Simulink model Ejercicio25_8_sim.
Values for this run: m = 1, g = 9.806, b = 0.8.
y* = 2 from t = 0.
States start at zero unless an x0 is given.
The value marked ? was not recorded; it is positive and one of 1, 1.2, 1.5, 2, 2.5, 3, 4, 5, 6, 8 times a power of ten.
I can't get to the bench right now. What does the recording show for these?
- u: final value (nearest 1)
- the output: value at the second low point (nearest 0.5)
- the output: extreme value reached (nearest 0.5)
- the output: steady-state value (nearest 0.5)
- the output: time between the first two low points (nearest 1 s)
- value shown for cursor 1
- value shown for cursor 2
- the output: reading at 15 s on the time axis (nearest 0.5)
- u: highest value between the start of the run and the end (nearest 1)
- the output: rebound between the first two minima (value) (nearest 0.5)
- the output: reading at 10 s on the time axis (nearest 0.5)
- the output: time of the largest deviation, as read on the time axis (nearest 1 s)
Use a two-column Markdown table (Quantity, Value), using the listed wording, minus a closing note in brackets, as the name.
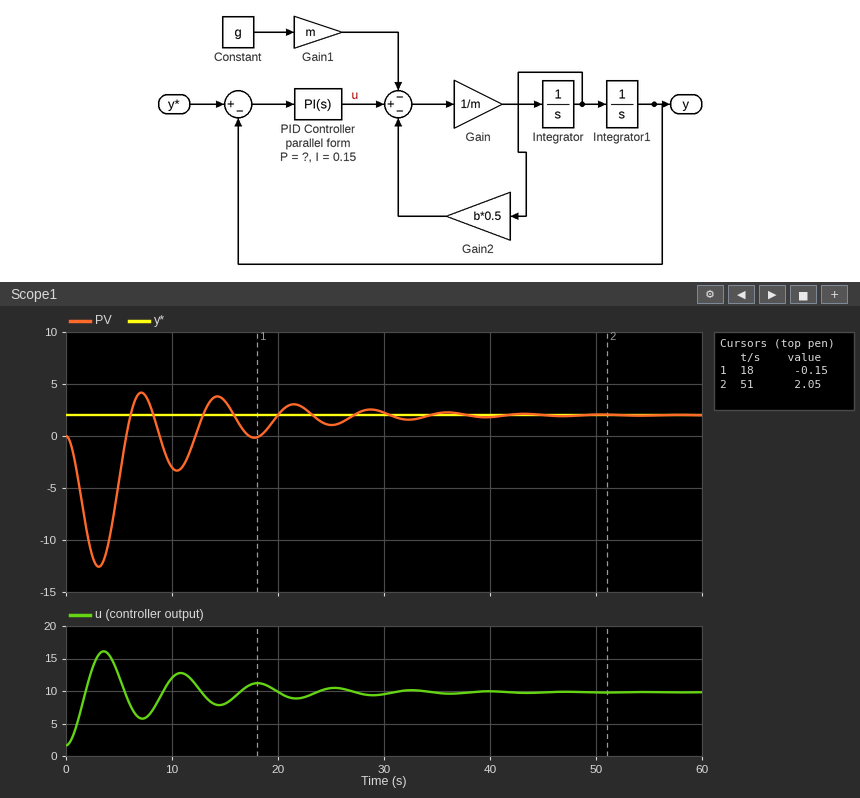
| Quantity | Value |
|---|---|
| u: final value | 10 |
| the output: value at the second low point | -3.5 |
| the output: extreme value reached | -12.5 |
| the output: steady-state value | 2.0 |
| the output: time between the first two low points | 7 s |
| value shown for cursor 1 | -0.15 |
| value shown for cursor 2 | 2.05 |
| the output: reading at 15 s on the time axis | 3.5 |
| u: highest value between the start of the run and the end | 16 |
| the output: rebound between the first two minima (value) | 4.0 |
| the output: reading at 10 s on the time axis | -3.0 |
| the output: time of the largest deviation, as read on the time axis | 3 s |
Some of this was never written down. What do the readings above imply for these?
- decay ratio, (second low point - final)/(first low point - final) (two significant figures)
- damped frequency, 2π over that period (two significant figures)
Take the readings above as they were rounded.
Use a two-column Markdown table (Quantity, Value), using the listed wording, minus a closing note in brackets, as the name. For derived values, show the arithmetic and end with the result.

| Quantity | Value |
|---|---|
| decay ratio, (second low point - final)/(first low point - final) | (-3.5 - 2) / (-12.5 - 2) = 0.38 |
| damped frequency, 2π over that period | 2π / 7 = 0.90 rad/s |
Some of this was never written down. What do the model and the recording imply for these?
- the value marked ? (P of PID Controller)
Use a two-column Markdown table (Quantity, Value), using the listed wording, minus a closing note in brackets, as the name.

| Quantity | Value |
|---|---|
| the value marked ? | 0.8 |
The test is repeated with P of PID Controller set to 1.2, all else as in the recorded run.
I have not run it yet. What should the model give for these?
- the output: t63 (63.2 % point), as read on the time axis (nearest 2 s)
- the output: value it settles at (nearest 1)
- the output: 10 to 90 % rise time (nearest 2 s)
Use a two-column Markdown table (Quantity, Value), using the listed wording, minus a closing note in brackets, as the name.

| Quantity | Value |
|---|---|
| the output: t63 (63.2 % point), as read on the time axis | 12 s |
| the output: value it settles at | 2 |
| the output: 10 to 90 % rise time | 18 s |
